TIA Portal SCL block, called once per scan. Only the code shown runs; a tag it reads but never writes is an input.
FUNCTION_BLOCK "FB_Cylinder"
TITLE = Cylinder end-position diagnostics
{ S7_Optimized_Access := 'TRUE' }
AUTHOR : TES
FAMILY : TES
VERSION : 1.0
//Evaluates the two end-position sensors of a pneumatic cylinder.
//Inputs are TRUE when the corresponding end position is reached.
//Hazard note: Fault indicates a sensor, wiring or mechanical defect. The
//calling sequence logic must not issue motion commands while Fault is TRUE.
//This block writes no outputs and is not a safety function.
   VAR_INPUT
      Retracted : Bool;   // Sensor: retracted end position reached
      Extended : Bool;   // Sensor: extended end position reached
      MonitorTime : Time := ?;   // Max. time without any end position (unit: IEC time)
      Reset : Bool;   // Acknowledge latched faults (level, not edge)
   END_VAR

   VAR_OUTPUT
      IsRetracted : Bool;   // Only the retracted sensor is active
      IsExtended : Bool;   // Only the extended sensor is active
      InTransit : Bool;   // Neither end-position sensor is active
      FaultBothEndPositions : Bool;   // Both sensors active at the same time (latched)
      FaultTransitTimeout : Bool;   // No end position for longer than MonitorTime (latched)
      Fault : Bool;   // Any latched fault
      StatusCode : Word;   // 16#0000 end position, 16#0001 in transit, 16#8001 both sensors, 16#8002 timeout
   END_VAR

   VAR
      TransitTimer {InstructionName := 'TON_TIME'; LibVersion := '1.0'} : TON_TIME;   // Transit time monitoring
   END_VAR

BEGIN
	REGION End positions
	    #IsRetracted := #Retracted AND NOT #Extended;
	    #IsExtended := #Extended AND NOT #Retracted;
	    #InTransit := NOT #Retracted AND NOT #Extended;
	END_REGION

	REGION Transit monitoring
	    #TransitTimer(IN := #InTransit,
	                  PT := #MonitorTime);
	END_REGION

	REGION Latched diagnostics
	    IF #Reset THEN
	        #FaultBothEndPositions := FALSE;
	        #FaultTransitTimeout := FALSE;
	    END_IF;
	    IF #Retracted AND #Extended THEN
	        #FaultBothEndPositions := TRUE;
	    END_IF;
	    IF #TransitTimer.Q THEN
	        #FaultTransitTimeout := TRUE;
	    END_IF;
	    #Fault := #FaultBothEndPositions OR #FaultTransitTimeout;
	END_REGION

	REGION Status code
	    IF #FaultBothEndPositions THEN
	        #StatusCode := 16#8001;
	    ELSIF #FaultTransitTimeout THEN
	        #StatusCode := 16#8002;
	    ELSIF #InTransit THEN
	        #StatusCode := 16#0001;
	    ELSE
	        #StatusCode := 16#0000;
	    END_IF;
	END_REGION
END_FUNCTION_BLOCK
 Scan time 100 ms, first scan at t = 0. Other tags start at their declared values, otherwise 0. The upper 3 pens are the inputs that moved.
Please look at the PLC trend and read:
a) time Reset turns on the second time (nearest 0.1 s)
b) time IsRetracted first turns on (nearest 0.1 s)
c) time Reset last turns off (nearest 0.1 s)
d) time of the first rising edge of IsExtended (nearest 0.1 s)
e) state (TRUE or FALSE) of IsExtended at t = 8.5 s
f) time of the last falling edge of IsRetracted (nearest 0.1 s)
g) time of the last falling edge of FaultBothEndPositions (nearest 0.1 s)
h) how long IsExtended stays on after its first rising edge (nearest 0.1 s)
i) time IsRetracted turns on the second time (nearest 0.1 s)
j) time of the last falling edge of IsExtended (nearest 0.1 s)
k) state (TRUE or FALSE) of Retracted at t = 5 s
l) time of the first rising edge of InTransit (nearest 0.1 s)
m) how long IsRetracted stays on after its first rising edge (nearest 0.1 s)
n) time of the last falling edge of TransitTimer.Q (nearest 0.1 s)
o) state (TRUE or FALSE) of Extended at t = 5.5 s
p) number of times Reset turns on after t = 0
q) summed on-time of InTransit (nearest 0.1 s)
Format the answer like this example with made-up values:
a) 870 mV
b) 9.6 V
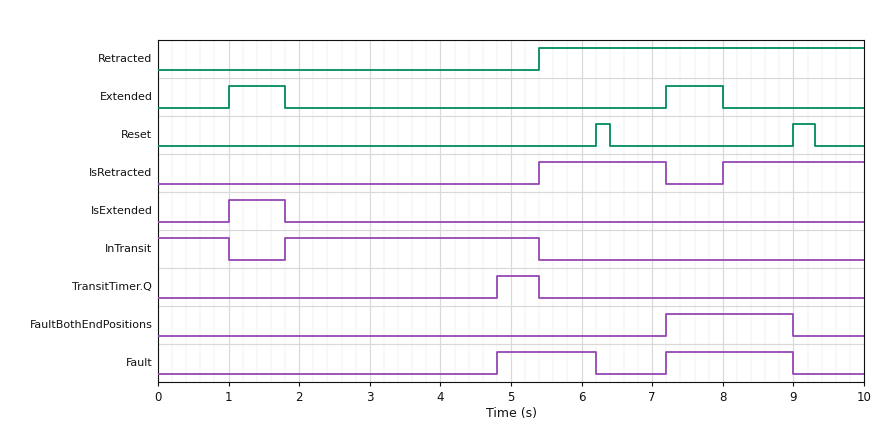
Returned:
a) 9.0 s
b) 5.4 s
c) 9.3 s
d) 1.0 s
e) FALSE
f) 7.2 s
g) 9.0 s
h) 0.8 s
i) 8.0 s
j) 1.8 s
k) FALSE
l) 1.8 s
m) 1.8 s
n) 5.4 s
o) FALSE
p) 2
q) 4.6 s
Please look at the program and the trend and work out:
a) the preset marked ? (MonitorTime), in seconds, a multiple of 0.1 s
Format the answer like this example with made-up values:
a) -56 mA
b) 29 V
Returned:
a) 3.0 s
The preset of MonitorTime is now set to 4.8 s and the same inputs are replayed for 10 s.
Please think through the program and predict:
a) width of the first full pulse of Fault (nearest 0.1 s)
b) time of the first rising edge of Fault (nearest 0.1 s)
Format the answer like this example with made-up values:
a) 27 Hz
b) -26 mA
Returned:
a) 1.8 s
b) 7.2 s
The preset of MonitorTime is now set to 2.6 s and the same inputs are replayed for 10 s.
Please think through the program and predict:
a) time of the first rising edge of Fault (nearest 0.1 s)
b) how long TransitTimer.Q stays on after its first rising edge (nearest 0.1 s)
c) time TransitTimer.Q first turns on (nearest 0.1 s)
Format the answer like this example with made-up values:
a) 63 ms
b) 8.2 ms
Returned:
a) 4.4 s
b) 1.0 s
c) 4.4 s
